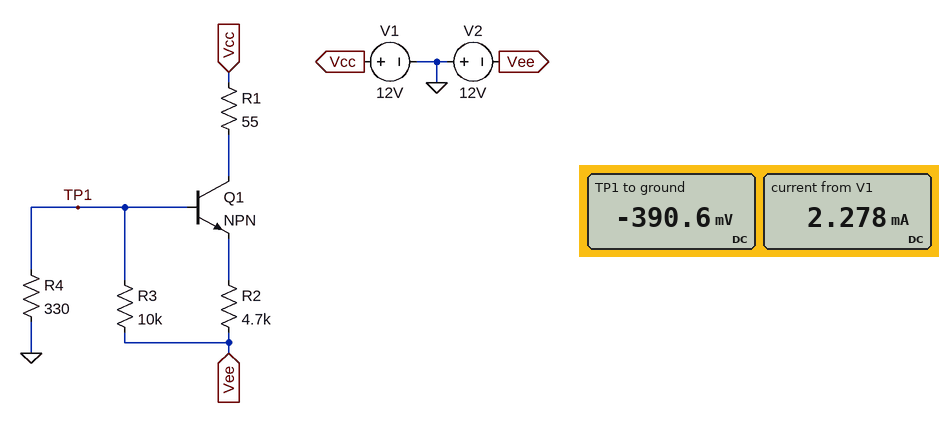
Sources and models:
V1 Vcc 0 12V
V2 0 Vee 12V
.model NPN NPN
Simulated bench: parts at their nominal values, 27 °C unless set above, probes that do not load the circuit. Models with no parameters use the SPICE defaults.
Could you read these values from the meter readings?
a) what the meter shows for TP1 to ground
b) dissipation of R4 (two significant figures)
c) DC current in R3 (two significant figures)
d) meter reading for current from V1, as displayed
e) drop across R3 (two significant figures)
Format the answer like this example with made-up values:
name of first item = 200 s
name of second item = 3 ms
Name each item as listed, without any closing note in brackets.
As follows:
what the meter shows for TP1 to ground = -390.6 mV
dissipation of R4 = 460 µW
DC current in R3 = 1.2 mA
meter reading for current from V1, as displayed = 2.278 mA
drop across R3 = 12 V
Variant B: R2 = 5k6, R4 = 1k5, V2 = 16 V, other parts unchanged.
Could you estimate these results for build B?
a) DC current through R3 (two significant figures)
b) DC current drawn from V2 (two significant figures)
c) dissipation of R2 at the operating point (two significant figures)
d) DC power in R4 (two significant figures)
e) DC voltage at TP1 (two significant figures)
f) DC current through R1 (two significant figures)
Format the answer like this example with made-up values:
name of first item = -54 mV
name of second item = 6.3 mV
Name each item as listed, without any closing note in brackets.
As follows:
DC current through R3 = 1.4 mA
DC current drawn from V2 = 3.7 mA
dissipation of R2 at the operating point = 31 mW
DC power in R4 = 3.0 mW
DC voltage at TP1 = -2.1 V
DC current through R1 = 2.3 mA
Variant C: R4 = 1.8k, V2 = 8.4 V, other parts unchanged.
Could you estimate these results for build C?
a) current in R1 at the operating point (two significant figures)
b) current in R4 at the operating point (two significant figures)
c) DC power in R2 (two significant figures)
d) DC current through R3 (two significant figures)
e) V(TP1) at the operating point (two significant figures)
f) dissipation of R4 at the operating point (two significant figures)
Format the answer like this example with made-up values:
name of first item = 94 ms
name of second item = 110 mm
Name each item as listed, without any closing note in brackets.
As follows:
current in R1 at the operating point = 1.3 mA
current in R4 at the operating point = 720 µA
DC power in R2 = 8.5 mW
DC current through R3 = 710 µA
V(TP1) at the operating point = -1.3 V
dissipation of R4 at the operating point = 940 µW
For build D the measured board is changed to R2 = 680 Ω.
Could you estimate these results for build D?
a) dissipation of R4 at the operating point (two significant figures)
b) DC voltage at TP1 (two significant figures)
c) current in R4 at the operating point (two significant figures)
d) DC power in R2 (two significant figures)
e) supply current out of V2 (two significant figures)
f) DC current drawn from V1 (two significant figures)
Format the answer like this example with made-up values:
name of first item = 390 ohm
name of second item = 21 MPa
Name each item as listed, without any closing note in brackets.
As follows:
dissipation of R4 at the operating point = 570 µW
DC voltage at TP1 = -430 mV
current in R4 at the operating point = 1.3 mA
DC power in R2 = 170 mW
supply current out of V2 = 17 mA
DC current drawn from V1 = 16 mA
